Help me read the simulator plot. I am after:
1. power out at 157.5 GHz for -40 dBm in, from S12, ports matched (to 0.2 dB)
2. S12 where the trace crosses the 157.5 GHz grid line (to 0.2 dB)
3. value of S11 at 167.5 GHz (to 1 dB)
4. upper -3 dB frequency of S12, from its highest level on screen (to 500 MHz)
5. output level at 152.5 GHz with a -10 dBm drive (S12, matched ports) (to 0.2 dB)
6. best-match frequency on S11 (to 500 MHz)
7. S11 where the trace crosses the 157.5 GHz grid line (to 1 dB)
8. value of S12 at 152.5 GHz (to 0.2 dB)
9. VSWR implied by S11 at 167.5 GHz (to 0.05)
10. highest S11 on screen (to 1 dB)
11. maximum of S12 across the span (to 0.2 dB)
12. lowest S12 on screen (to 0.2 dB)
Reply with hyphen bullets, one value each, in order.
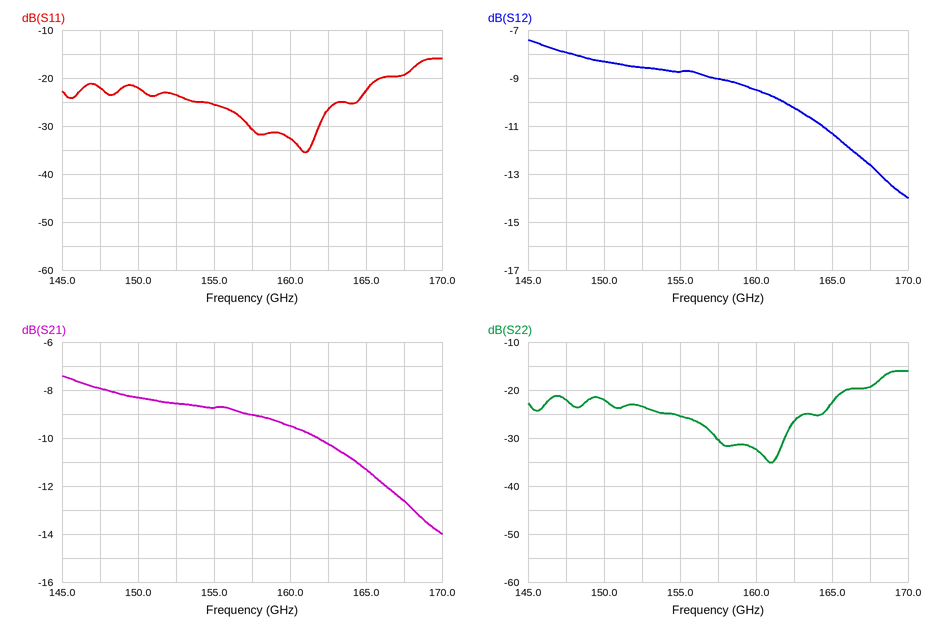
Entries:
- -49.0 dBm
- -9.0 dB
- -19 dB
- 163.0 GHz
- -18.6 dBm
- 161.0 GHz
- -31 dB
- -8.6 dB
- 1.25
- -16 dB
- -7.4 dB
- -14.0 dB
